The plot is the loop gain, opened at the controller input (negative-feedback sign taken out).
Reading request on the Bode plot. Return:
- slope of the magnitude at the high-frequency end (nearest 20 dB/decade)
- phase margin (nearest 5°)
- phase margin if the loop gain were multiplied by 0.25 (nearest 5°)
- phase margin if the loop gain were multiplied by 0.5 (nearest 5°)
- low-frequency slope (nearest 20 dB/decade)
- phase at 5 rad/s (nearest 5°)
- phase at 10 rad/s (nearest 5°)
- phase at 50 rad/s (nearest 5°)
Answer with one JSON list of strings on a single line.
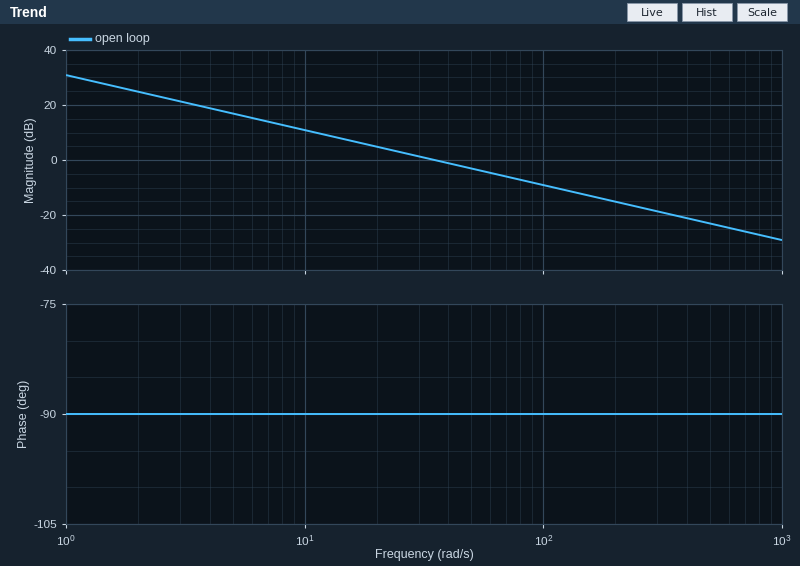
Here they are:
["-20 dB/decade", "90°", "90°", "90°", "-20 dB/decade", "-90°", "-90°", "-90°"]
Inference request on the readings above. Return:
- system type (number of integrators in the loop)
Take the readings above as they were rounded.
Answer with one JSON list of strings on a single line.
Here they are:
["1"]
